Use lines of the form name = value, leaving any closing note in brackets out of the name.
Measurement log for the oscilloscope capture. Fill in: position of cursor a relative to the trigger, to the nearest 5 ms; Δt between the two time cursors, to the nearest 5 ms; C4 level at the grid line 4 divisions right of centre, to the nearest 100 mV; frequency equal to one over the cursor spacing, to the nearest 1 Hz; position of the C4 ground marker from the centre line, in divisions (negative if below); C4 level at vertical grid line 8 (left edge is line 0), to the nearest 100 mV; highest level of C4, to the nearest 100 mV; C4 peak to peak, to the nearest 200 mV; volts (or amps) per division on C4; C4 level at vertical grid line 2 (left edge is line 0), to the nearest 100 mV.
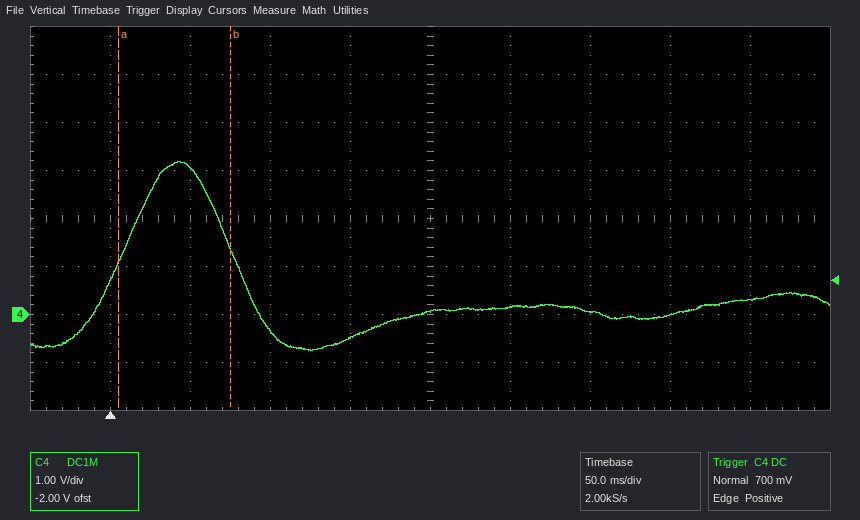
position of cursor a relative to the trigger, to the nearest 5 ms = +5 ms
Δt between the two time cursors, to the nearest 5 ms = 70 ms
C4 level at the grid line 4 divisions right of centre, to the nearest 100 mV = 300 mV
frequency equal to one over the cursor spacing, to the nearest 1 Hz = 14 Hz
position of the C4 ground marker from the centre line, in divisions = -2.0 div
C4 level at vertical grid line 8 (left edge is line 0), to the nearest 100 mV = 0.0 V
highest level of C4, to the nearest 100 mV = 3.2 V
C4 peak to peak, to the nearest 200 mV = 4.0 V
volts (or amps) per division on C4 = 1 V
C4 level at vertical grid line 2 (left edge is line 0), to the nearest 100 mV = 3.1 V
